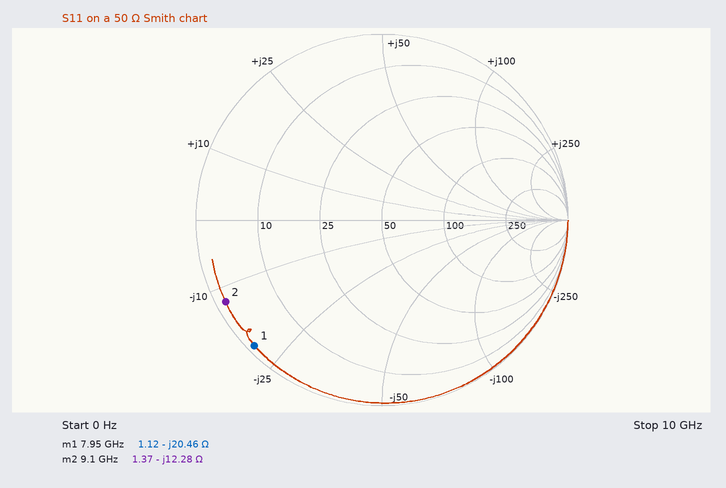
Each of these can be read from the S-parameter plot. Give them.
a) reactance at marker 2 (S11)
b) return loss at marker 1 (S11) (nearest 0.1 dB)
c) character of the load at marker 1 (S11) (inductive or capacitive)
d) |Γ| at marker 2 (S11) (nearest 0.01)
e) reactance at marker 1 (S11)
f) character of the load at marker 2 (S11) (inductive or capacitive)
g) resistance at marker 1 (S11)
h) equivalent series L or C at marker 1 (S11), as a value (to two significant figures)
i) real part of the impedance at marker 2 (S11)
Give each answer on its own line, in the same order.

-12.28 Ω
0.3 dB
capacitive
0.95
-20.46 Ω
capacitive
1.12 Ω
980 fF
1.37 Ω
